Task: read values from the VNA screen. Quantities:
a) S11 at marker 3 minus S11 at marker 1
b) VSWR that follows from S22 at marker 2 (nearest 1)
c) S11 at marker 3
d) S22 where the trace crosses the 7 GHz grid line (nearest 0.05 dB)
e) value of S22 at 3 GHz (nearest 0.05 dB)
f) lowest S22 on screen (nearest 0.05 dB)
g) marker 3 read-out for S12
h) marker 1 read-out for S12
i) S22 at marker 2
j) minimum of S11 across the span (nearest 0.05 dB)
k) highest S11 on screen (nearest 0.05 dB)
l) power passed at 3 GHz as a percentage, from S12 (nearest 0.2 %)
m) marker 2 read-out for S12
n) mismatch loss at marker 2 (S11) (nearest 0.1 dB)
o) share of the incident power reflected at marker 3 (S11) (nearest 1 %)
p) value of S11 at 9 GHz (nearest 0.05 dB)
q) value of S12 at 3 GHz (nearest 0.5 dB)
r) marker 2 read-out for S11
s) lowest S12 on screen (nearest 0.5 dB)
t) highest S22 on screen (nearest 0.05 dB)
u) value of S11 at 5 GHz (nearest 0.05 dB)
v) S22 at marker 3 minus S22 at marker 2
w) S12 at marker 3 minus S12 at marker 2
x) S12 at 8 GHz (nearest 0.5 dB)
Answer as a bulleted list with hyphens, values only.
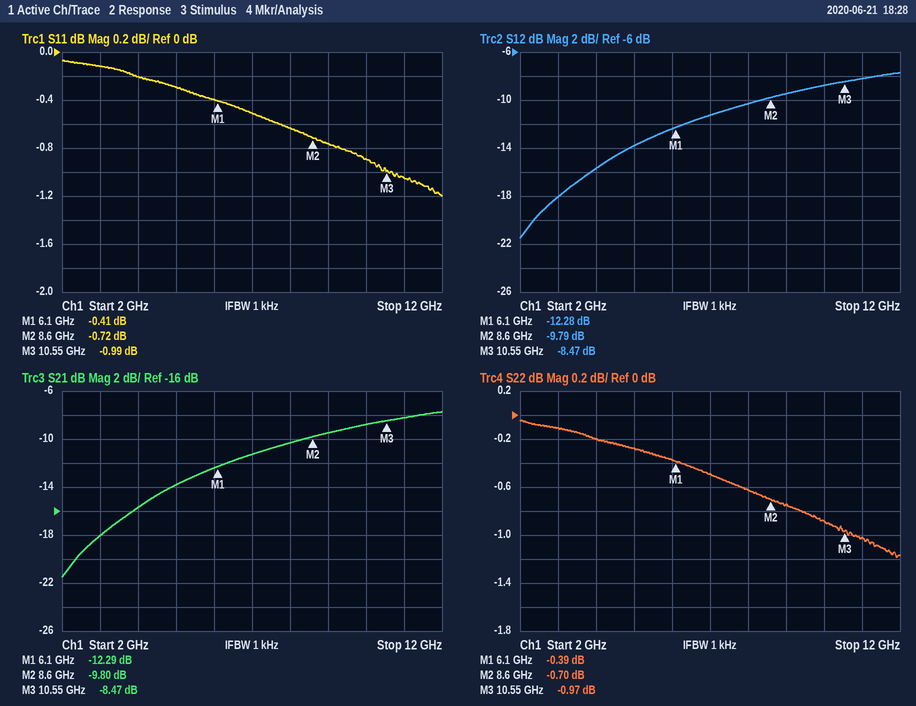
- -0.58 dB
- 25
- -0.99 dB
- -0.50 dB
- -0.10 dB
- -1.20 dB
- -8.47 dB
- -12.28 dB
- -0.70 dB
- -1.20 dB
- -0.05 dB
- 1.6 %
- -9.79 dB
- 8.2 dB
- 80 %
- -0.75 dB
- -18.0 dB
- -0.72 dB
- -21.5 dB
- -0.05 dB
- -0.30 dB
- -0.27 dB
- 1.32 dB
- -10.5 dB
